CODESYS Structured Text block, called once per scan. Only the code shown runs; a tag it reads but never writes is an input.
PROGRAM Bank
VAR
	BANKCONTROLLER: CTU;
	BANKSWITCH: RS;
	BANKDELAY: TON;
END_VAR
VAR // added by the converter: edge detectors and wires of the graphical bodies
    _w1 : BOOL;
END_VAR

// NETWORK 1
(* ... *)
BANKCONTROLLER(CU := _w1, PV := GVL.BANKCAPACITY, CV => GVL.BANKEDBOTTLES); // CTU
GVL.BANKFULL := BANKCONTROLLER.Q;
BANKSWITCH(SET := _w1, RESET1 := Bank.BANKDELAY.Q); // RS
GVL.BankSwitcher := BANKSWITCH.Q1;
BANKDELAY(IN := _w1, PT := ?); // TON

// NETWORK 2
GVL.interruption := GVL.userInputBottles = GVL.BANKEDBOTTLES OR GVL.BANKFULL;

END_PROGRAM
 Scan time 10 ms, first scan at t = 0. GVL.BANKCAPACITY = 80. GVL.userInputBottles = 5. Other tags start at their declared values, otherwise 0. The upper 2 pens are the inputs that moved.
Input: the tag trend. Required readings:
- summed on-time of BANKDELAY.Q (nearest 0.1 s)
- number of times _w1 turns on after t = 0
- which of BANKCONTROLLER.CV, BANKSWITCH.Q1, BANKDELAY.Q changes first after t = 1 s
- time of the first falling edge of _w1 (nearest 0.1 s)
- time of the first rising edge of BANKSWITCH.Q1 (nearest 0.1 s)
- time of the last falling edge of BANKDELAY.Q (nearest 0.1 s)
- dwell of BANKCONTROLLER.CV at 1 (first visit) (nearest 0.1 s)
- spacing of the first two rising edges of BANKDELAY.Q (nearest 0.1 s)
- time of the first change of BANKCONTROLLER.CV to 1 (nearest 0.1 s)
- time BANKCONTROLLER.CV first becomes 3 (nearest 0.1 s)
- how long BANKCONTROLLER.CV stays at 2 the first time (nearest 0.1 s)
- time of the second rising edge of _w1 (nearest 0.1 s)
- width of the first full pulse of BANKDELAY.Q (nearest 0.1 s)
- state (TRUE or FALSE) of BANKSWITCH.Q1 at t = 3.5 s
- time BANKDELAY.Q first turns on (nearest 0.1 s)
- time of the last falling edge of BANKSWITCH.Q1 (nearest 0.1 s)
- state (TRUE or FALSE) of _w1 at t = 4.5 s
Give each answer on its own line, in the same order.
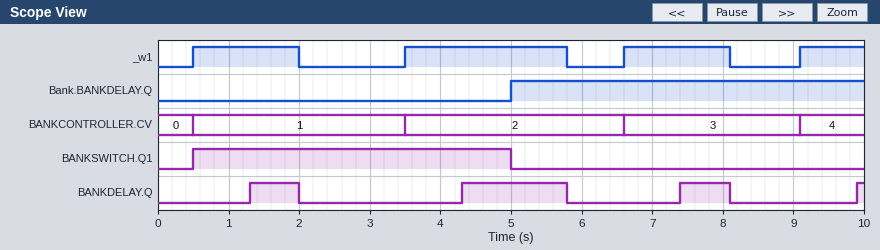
3.0 s
4
BANKDELAY.Q
2.0 s
0.5 s
8.1 s
3.0 s
3.0 s
0.5 s
6.6 s
3.1 s
3.5 s
0.7 s
TRUE
1.3 s
5.0 s
TRUE
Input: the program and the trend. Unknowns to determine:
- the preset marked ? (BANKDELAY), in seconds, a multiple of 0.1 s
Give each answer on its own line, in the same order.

0.8 s
